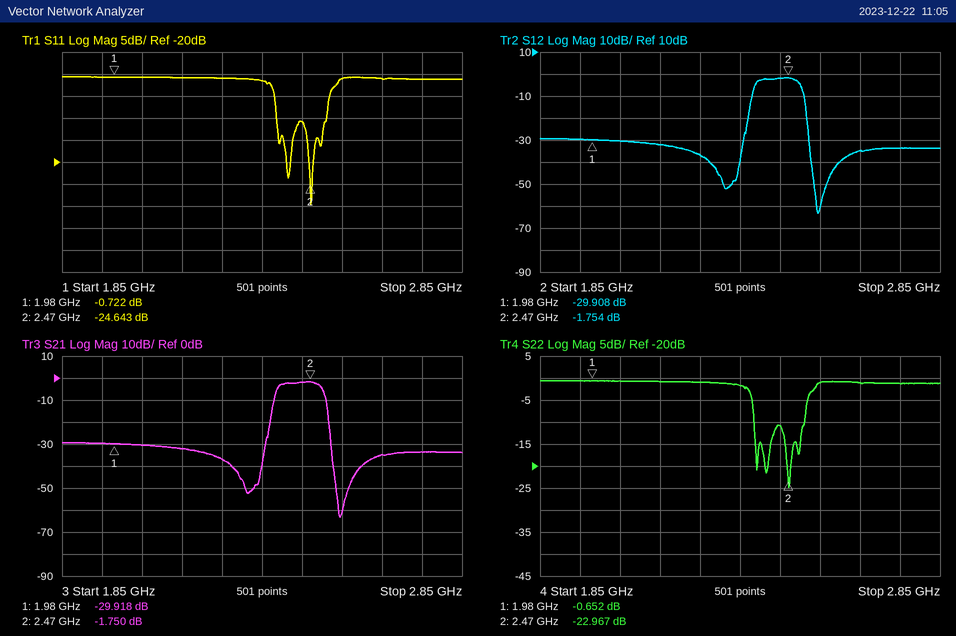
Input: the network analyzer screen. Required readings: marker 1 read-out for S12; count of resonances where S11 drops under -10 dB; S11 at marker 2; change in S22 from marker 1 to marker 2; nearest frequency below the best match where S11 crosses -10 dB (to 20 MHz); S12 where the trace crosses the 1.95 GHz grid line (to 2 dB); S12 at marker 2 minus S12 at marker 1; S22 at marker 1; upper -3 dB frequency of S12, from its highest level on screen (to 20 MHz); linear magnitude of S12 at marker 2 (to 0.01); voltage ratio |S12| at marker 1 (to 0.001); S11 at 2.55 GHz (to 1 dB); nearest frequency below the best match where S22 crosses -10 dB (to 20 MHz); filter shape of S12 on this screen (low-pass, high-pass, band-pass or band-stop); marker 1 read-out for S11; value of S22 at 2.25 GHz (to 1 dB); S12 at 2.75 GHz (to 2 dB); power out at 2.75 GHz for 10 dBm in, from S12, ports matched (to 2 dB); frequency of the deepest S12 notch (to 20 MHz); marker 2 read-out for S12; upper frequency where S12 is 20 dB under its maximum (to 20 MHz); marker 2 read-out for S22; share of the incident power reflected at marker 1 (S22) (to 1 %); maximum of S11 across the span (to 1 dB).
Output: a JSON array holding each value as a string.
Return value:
["-29.908 dB", "2", "-24.643 dB", "-22.315 dB", "2.38 GHz", "-30 dB", "28.154 dB", "-0.652 dB", "2.50 GHz", "0.82", "0.032", "-1 dB", "2.38 GHz", "band-pass", "-0.722 dB", "-1 dB", "-34 dB", "-24 dBm", "2.54 GHz", "-1.754 dB", "2.52 GHz", "-22.967 dB", "86 %", "-1 dB"]
